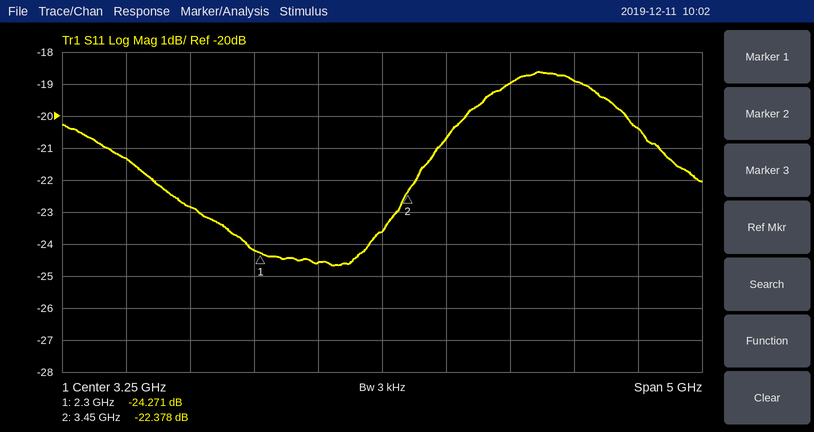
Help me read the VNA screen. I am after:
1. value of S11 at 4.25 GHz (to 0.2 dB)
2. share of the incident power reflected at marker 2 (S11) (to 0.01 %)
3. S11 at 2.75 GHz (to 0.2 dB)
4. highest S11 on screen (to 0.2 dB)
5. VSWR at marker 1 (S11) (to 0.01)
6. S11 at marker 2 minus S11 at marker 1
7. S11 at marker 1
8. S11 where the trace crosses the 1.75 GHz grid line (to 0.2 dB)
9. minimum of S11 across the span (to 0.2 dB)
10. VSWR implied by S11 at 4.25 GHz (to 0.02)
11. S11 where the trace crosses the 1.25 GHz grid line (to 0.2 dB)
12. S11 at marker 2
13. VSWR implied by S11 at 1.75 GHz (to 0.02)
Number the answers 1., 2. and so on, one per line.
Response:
1. -19.0 dB
2. 0.58 %
3. -24.6 dB
4. -18.6 dB
5. 1.13
6. 1.893 dB
7. -24.271 dB
8. -22.8 dB
9. -24.6 dB
10. 1.26
11. -21.4 dB
12. -22.378 dB
13. 1.16
